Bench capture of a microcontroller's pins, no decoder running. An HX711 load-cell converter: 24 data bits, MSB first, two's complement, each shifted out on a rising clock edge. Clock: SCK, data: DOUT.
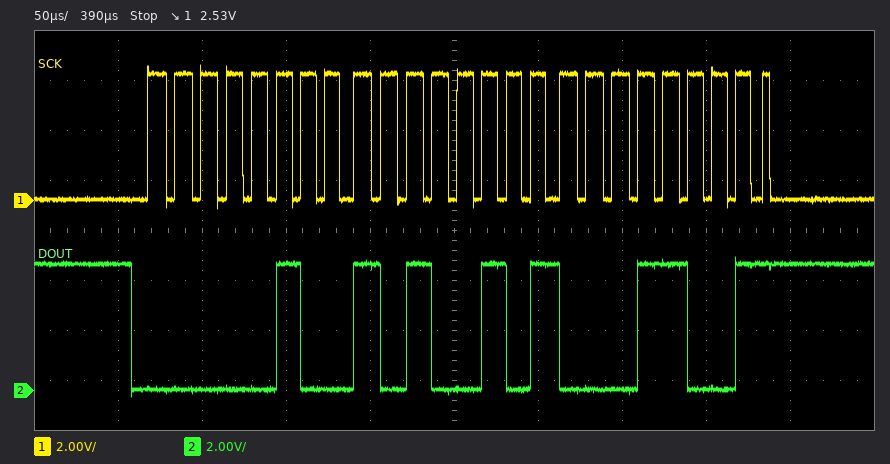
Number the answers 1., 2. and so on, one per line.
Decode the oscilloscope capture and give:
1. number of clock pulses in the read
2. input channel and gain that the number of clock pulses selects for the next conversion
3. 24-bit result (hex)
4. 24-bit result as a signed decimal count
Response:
1. 25
2. channel A, gain 128
3. 0x04A519
4. 304409
